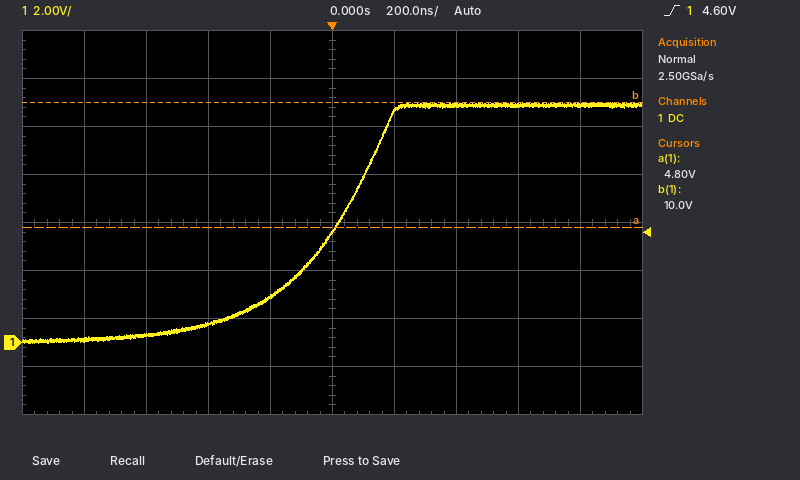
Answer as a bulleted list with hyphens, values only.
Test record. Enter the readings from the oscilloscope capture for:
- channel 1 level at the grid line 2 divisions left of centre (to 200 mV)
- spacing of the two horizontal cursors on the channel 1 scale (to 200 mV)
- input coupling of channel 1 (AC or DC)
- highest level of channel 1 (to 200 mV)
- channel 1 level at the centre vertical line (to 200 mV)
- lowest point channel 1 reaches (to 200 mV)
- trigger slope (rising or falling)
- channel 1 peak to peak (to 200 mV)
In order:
- 800 mV
- 5.2 V
- DC
- 10.0 V
- 4.6 V
- 0.0 V
- rising
- 10.0 V
